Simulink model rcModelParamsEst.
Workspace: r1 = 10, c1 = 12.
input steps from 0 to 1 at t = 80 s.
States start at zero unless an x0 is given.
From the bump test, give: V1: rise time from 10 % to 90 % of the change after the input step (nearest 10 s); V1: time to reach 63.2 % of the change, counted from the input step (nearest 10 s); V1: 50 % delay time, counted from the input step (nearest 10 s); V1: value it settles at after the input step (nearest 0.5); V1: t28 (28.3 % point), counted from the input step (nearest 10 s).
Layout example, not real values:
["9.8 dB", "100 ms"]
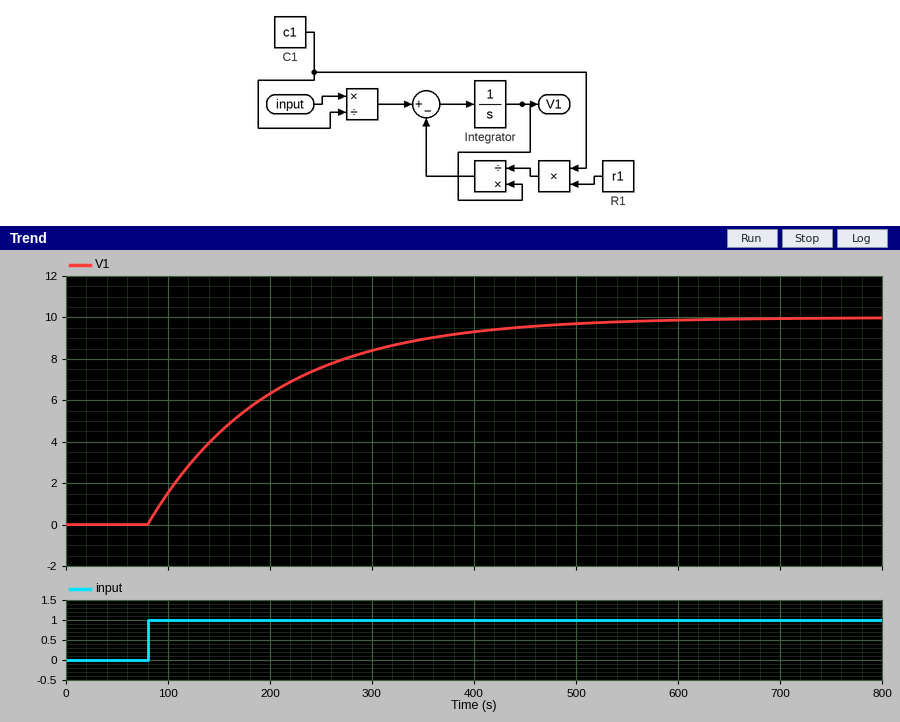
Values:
["260 s", "120 s", "80 s", "10.0", "40 s"]
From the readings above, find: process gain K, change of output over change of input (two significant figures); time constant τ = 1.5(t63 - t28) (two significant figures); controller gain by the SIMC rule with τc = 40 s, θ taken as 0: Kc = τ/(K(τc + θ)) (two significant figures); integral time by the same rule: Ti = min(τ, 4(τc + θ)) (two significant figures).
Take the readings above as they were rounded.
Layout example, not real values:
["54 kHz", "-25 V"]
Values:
["10", "120 s", "0.30", "120 s"]
